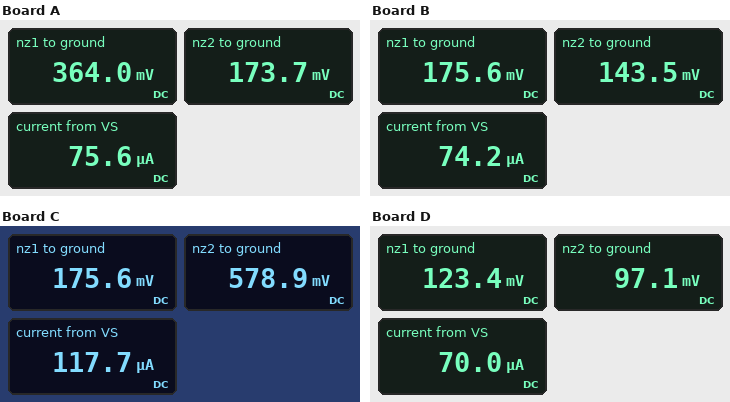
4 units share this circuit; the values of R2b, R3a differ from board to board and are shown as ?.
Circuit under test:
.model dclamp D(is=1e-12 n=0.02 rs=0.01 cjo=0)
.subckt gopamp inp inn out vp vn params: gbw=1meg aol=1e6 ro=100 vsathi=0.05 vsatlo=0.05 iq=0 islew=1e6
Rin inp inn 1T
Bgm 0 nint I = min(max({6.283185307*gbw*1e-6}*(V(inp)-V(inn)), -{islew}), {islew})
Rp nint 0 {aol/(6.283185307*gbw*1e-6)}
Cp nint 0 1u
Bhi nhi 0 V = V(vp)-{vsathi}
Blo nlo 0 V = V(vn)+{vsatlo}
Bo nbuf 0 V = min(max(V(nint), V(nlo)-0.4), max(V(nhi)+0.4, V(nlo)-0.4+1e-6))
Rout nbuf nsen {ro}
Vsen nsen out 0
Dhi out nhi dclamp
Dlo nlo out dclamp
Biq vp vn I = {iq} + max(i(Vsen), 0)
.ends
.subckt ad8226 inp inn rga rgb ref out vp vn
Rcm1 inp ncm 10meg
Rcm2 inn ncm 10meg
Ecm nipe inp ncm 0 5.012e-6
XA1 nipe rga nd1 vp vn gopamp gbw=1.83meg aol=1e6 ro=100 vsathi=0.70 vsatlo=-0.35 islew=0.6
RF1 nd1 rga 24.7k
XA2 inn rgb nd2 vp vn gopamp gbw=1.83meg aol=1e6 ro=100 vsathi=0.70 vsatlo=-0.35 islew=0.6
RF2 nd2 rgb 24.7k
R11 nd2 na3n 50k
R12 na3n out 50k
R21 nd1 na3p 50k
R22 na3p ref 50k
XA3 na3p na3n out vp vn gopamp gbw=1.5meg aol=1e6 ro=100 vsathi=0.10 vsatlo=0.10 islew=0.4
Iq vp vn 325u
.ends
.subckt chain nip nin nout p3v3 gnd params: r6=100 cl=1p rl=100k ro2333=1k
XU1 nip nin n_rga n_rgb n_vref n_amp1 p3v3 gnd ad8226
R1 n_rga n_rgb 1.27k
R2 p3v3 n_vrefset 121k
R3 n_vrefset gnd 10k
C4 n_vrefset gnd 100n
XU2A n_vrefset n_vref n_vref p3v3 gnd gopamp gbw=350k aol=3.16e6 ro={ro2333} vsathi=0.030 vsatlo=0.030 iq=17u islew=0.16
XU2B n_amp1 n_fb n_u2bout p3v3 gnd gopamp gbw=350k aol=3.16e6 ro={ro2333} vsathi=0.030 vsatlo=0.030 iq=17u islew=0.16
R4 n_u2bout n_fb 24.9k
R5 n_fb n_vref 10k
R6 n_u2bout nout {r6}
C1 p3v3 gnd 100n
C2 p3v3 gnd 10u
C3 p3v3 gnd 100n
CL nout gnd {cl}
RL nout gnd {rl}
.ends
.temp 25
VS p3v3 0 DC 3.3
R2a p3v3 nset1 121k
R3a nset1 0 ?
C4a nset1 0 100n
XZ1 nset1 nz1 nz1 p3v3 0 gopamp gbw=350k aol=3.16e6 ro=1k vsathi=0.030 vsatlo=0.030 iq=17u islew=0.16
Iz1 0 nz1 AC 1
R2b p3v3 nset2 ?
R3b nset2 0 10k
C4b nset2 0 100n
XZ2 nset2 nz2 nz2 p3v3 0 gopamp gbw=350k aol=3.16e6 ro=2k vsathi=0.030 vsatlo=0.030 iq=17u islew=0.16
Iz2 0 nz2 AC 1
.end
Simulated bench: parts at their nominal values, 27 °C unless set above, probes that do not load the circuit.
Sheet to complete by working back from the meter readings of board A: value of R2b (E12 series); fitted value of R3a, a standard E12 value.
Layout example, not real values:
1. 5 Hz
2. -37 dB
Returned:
1. 180 kΩ
2. 15 kΩ
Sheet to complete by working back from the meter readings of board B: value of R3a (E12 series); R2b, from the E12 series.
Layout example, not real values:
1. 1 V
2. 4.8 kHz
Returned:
1. 6.8 kΩ
2. 220 kΩ
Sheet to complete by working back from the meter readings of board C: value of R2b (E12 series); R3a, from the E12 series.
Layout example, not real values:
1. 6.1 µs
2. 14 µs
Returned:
1. 47 kΩ
2. 6.8 kΩ
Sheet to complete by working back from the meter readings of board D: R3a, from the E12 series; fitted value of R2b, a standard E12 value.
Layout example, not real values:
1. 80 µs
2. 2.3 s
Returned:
1. 4.7 kΩ
2. 330 kΩ
